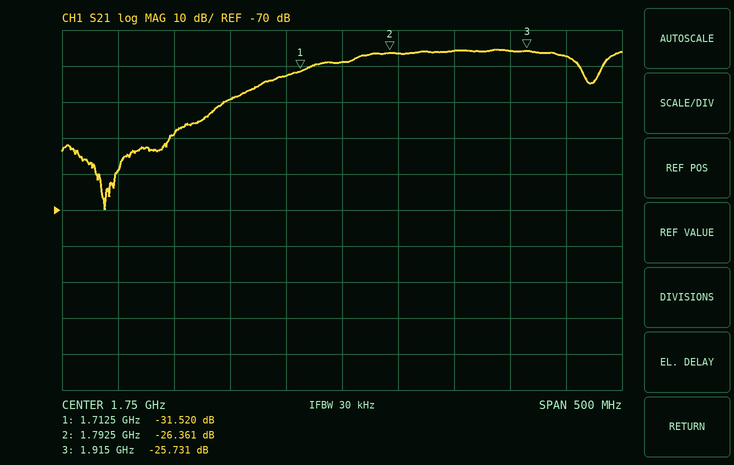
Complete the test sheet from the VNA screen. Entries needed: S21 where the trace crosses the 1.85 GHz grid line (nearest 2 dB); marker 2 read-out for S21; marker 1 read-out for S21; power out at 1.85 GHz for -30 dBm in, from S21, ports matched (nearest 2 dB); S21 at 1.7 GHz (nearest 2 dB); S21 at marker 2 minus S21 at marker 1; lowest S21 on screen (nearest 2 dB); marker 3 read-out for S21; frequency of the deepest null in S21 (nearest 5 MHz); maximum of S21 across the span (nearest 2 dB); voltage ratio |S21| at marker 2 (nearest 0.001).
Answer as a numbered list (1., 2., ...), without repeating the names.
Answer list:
1. -26 dB
2. -26.361 dB
3. -31.520 dB
4. -56 dBm
5. -32 dB
6. 5.159 dB
7. -70 dB
8. -25.731 dB
9. 1.540 GHz
10. -26 dB
11. 0.048
